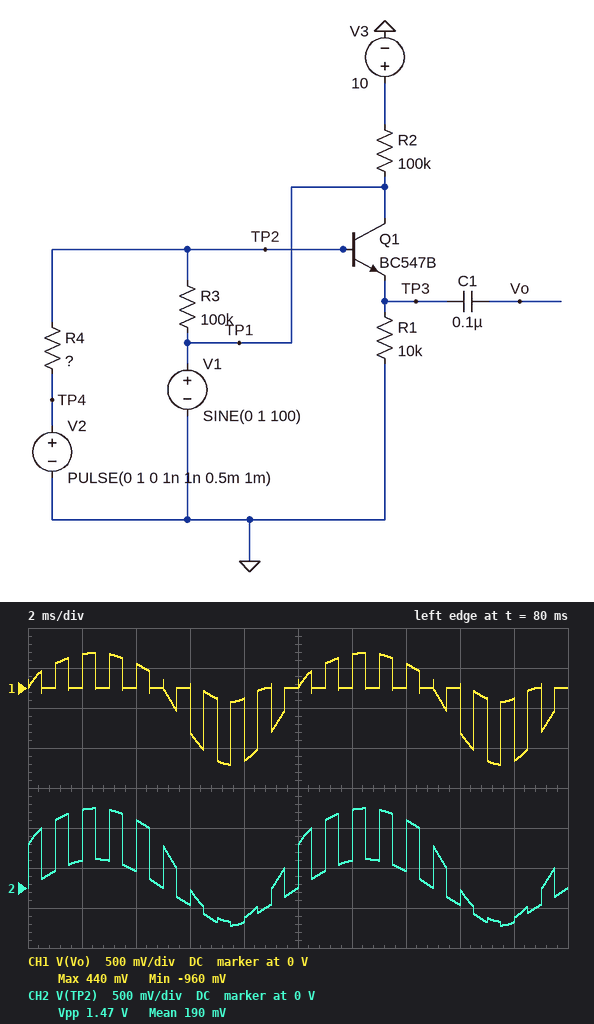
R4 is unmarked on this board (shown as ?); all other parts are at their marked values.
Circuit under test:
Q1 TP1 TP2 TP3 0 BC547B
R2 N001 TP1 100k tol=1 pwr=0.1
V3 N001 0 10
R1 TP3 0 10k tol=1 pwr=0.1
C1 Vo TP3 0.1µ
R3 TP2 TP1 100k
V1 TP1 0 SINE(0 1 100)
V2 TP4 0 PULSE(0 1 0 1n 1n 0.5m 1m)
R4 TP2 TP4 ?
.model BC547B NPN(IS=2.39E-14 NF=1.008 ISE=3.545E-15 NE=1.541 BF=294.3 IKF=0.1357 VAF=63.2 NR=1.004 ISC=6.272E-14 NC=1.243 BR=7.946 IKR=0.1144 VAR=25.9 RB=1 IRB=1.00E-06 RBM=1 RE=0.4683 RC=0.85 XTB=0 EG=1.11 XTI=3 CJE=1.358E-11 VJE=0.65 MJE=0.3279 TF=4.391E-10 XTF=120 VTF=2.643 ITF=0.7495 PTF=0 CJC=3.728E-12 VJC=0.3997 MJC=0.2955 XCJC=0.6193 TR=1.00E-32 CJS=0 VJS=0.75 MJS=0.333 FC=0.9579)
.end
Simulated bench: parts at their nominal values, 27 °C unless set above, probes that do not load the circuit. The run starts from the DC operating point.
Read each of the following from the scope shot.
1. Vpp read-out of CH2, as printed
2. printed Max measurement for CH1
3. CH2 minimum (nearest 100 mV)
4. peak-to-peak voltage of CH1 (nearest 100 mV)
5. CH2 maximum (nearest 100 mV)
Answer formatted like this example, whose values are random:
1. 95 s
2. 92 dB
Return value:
1. 1.47 V
2. 440 mV
3. -500 mV
4. 1.4 V
5. 1.0 V
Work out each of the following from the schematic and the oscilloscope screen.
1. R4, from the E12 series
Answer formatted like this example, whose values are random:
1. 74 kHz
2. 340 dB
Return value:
1. 56 kΩ
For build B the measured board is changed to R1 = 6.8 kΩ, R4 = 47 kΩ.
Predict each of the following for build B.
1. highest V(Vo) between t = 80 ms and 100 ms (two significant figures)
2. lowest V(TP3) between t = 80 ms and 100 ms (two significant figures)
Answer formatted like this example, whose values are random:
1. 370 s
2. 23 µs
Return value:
1. 430 mV
2. -930 mV
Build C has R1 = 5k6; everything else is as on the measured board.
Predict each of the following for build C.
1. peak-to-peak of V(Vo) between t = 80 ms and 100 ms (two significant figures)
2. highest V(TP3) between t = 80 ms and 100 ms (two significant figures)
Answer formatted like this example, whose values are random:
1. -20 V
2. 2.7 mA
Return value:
1. 1.1 V
2. 420 mV
